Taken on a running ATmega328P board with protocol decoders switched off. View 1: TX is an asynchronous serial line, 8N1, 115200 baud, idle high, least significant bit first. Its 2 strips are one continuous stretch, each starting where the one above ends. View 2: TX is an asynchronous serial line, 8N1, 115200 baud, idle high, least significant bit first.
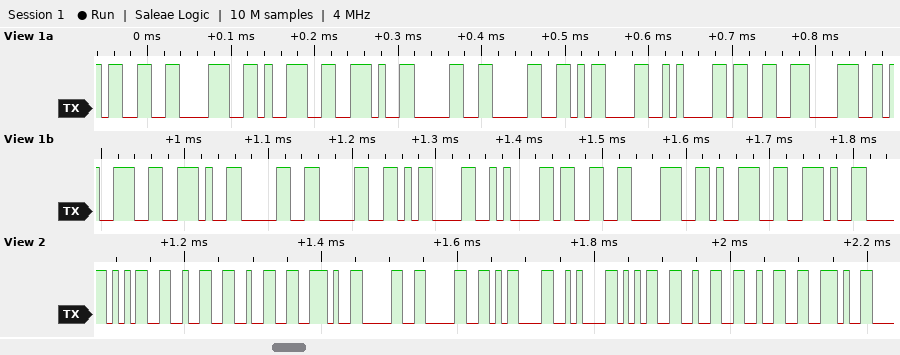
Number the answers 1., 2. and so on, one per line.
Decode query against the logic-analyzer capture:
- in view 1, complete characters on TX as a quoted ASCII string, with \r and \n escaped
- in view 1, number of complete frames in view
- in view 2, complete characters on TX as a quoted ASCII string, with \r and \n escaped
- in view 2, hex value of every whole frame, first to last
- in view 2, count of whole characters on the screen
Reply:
1. "389.00\r\n389.00\r\n389."
2. 20
3. "522.00\r\n522."
4. 35 32 32 2E 30 30 0D 0A 35 32 32 2E
5. 12
